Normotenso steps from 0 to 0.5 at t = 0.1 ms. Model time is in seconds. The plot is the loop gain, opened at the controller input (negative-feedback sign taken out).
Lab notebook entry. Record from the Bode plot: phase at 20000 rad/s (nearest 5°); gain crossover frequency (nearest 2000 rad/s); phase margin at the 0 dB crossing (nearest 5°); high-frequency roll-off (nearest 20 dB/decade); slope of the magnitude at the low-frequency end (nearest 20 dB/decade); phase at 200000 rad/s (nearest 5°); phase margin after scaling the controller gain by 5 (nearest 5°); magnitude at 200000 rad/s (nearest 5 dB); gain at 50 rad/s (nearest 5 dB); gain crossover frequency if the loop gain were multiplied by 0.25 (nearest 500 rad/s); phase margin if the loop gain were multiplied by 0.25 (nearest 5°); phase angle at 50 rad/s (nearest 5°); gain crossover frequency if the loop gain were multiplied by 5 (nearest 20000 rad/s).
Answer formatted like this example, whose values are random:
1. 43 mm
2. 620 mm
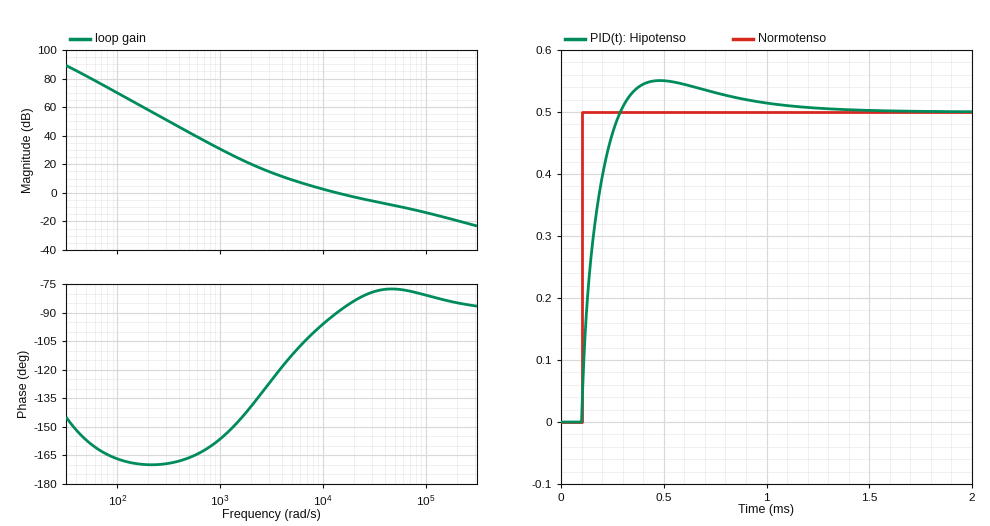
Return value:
1. -85°
2. 14000 rad/s
3. 90°
4. -20 dB/decade
5. -40 dB/decade
6. -85°
7. 100°
8. -20 dB
9. 80 dB
10. 4000 rad/s
11. 60°
12. -155°
13. 100000 rad/s
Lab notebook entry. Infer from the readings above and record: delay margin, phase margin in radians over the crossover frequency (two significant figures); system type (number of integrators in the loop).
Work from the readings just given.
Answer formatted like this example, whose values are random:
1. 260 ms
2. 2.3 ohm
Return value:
1. 0.00011 s
2. 2
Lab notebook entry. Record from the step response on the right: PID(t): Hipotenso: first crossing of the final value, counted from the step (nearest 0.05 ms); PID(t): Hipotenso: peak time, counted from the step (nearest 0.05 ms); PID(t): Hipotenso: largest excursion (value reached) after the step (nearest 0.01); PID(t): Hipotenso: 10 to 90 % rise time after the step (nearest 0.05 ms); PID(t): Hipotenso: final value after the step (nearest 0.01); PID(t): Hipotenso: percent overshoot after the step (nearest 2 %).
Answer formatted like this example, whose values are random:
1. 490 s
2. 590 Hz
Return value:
1. 0.20 ms
2. 0.40 ms
3. 0.55
4. 0.15 ms
5. 0.50
6. 10 %
